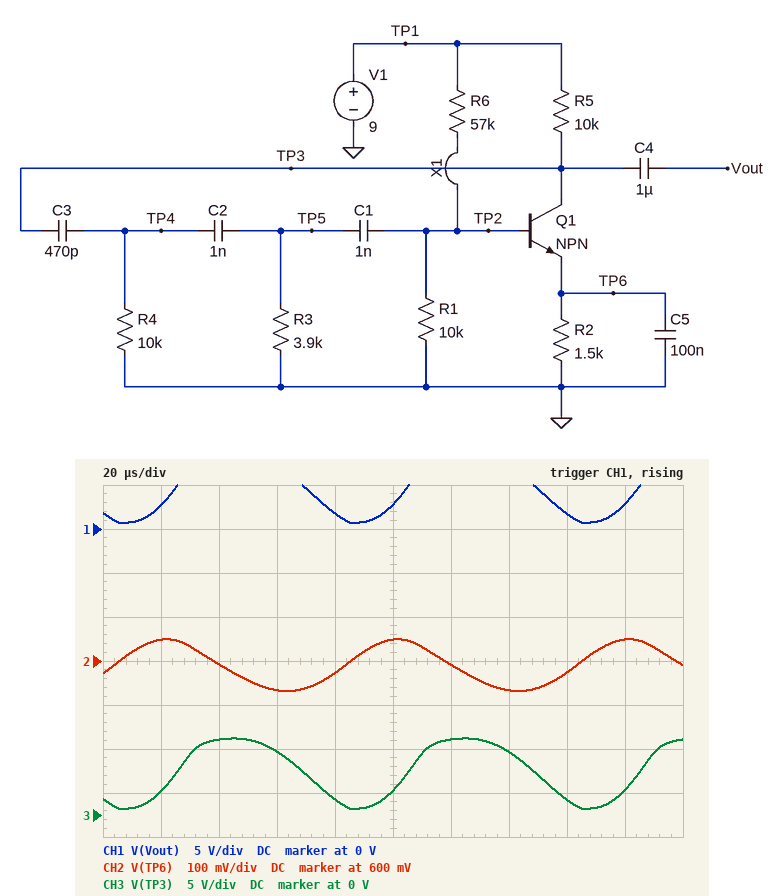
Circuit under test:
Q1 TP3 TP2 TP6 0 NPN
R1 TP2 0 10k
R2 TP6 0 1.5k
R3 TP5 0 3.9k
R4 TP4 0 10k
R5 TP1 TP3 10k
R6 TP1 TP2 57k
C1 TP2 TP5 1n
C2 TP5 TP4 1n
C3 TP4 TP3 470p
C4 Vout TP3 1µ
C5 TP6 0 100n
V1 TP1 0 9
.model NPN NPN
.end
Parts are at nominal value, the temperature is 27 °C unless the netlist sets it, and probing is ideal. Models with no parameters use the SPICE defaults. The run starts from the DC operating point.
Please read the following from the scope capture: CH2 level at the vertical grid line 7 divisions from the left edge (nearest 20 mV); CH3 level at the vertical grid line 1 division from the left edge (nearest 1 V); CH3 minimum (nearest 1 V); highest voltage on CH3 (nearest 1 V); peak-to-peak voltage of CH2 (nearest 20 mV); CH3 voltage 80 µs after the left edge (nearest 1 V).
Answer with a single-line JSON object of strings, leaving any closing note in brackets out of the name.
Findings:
{"CH2 level at the vertical grid line 7 divisions from the left edge": "540 mV", "CH3 level at the vertical grid line 1 division from the left edge": "3 V", "CH3 minimum": "1 V", "highest voltage on CH3": "9 V", "peak-to-peak voltage of CH2": "120 mV", "CH3 voltage 80 µs after the left edge": "2 V"}
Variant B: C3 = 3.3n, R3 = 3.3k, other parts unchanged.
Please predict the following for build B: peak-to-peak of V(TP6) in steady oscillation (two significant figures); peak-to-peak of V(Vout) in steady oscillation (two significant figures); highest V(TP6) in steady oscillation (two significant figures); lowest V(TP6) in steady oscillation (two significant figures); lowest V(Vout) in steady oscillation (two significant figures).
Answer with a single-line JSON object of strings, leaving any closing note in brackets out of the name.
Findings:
{"peak-to-peak of V(TP6) in steady oscillation": "150 mV", "peak-to-peak of V(Vout) in steady oscillation": "4.9 V", "highest V(TP6) in steady oscillation": "660 mV", "lowest V(TP6) in steady oscillation": "510 mV", "lowest V(Vout) in steady oscillation": "2.6 V"}
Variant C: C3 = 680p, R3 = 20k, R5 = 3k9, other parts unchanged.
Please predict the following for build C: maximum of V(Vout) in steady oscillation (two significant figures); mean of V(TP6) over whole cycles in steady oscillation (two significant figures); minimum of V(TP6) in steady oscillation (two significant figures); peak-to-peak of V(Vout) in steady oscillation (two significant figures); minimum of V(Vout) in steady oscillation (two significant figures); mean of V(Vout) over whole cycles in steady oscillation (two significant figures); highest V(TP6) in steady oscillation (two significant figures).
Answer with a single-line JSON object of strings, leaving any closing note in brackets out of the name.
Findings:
{"maximum of V(Vout) in steady oscillation": "8.9 V", "mean of V(TP6) over whole cycles in steady oscillation": "580 mV", "minimum of V(TP6) in steady oscillation": "520 mV", "peak-to-peak of V(Vout) in steady oscillation": "2.9 V", "minimum of V(Vout) in steady oscillation": "6.0 V", "mean of V(Vout) over whole cycles in steady oscillation": "7.5 V", "highest V(TP6) in steady oscillation": "640 mV"}
